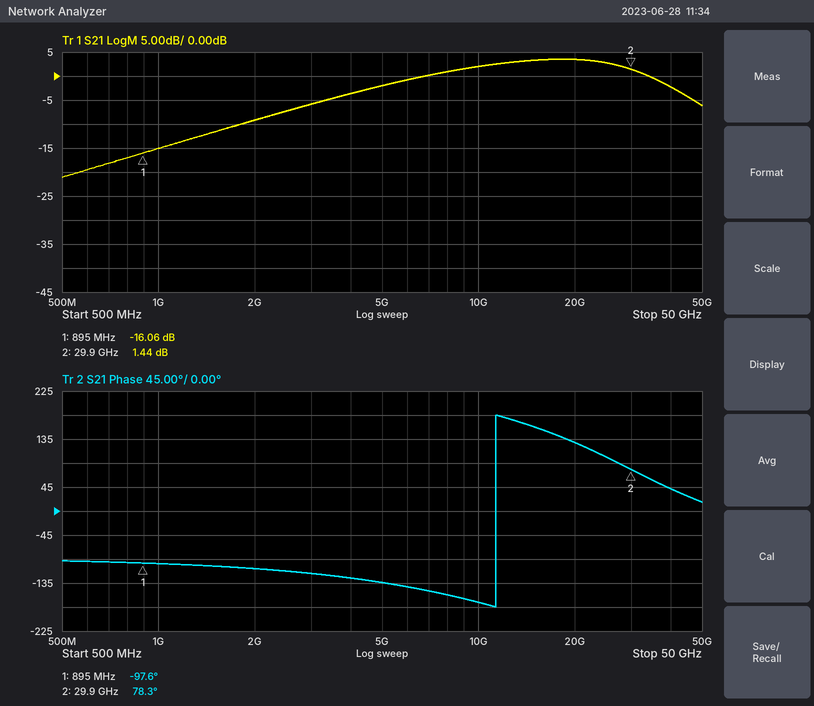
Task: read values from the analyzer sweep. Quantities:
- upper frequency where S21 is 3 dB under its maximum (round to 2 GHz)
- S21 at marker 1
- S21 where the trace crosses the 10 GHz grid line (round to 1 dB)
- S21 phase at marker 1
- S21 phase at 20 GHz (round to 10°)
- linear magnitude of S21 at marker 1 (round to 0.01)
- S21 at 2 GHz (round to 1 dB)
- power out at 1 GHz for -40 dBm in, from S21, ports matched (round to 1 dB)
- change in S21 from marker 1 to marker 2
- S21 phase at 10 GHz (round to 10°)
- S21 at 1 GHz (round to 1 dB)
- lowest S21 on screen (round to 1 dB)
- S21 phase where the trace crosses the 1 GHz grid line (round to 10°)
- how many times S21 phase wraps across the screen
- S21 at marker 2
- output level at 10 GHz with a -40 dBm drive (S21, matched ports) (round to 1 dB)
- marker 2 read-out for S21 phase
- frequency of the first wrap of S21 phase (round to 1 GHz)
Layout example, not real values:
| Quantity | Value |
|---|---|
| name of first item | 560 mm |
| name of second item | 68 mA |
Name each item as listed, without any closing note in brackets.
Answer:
| Quantity | Value |
|---|---|
| upper frequency where S21 is 3 dB under its maximum | 32 GHz |
| S21 at marker 1 | -16.06 dB |
| S21 where the trace crosses the 10 GHz grid line | 2 dB |
| S21 phase at marker 1 | -97.6° |
| S21 phase at 20 GHz | 130° |
| linear magnitude of S21 at marker 1 | 0.16 |
| S21 at 2 GHz | -9 dB |
| power out at 1 GHz for -40 dBm in, from S21, ports matched | -55 dBm |
| change in S21 from marker 1 to marker 2 | 17.50 dB |
| S21 phase at 10 GHz | -170° |
| S21 at 1 GHz | -15 dB |
| lowest S21 on screen | -21 dB |
| S21 phase where the trace crosses the 1 GHz grid line | -100° |
| how many times S21 phase wraps across the screen | 1 |
| S21 at marker 2 | 1.44 dB |
| output level at 10 GHz with a -40 dBm drive (S21, matched ports) | -38 dBm |
| marker 2 read-out for S21 phase | 78.3° |
| frequency of the first wrap of S21 phase | 11 GHz |
